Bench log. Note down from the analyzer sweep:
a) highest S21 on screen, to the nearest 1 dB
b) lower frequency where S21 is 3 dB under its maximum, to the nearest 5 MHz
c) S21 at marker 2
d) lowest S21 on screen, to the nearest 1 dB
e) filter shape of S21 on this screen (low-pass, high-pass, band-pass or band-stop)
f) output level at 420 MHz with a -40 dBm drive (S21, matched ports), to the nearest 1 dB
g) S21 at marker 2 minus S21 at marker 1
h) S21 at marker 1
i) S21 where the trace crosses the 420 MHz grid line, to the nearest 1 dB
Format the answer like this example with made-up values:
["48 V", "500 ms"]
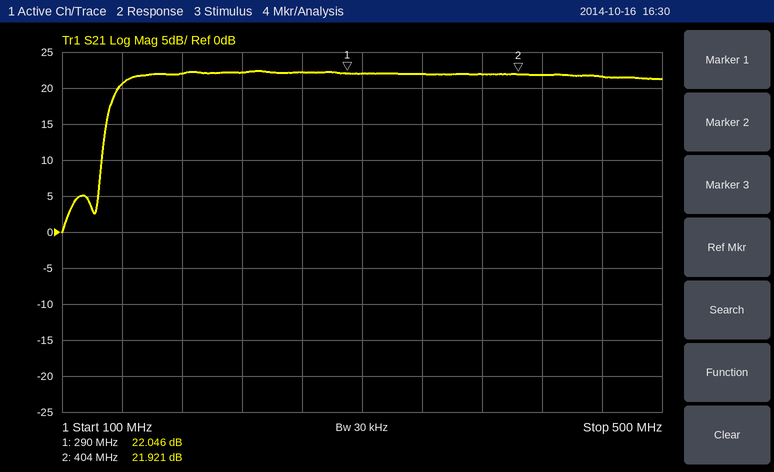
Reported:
["22 dB", "135 MHz", "21.921 dB", "0 dB", "high-pass", "-18 dBm", "-0.125 dB", "22.046 dB", "22 dB"]
